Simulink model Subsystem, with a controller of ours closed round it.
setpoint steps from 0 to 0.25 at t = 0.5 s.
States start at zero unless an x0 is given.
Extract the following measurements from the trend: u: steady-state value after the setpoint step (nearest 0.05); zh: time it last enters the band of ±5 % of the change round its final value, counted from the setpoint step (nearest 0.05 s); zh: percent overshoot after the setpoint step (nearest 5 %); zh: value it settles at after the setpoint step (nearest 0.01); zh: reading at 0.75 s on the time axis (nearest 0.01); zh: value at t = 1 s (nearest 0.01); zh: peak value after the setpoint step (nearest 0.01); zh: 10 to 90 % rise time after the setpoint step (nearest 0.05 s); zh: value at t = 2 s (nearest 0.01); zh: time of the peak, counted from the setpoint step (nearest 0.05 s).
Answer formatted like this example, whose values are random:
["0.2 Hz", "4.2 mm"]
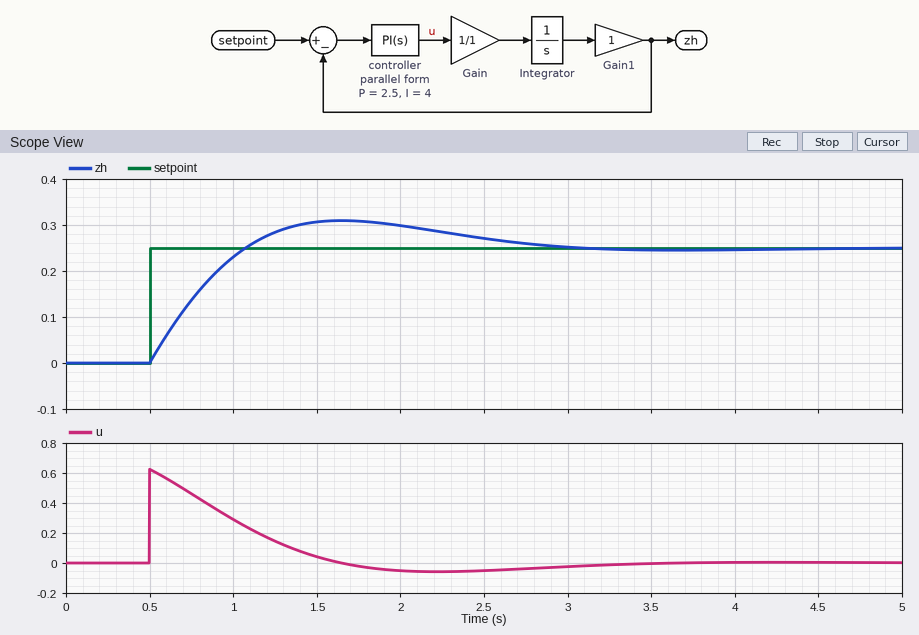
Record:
["0.00", "2.20 s", "25 %", "0.25", "0.14", "0.23", "0.31", "0.45 s", "0.30", "1.15 s"]
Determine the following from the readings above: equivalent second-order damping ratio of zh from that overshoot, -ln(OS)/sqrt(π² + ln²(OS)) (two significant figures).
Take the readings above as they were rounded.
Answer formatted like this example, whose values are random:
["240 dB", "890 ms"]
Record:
["0.40"]
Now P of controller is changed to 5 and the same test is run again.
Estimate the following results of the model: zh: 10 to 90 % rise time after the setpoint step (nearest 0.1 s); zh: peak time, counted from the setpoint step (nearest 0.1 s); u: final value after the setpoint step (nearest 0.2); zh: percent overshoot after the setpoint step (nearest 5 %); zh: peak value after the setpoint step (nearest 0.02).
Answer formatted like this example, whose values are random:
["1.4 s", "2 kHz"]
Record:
["0.3 s", "0.9 s", "0.0", "10 %", "0.28"]
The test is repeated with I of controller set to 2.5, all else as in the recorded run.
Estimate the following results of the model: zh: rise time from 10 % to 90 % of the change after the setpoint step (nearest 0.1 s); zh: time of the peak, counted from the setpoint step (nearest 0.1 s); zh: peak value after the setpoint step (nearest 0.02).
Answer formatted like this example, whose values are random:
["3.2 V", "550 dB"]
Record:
["0.5 s", "1.4 s", "0.30"]
